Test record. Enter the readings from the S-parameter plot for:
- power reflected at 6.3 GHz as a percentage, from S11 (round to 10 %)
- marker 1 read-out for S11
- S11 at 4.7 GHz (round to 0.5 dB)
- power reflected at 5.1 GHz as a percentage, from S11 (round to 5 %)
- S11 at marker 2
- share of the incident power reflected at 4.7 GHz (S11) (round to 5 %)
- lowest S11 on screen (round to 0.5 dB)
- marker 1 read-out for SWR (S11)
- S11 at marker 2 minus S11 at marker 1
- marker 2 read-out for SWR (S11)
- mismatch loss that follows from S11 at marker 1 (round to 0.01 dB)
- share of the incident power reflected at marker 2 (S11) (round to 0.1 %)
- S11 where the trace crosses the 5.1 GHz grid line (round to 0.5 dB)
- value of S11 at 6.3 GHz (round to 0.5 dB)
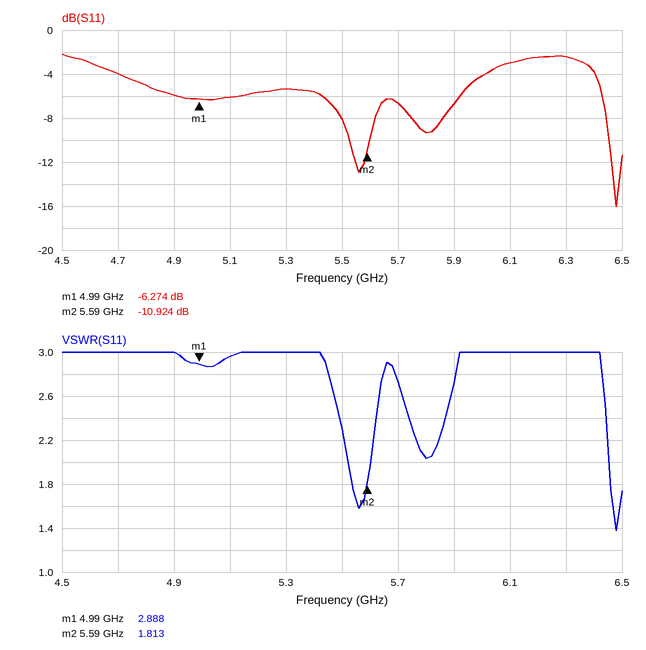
60 %
-6.274 dB
-4.0 dB
25 %
-10.924 dB
40 %
-16.0 dB
2.888
-4.650 dB
1.813
1.17 dB
8.1 %
-6.0 dB
-2.5 dB
